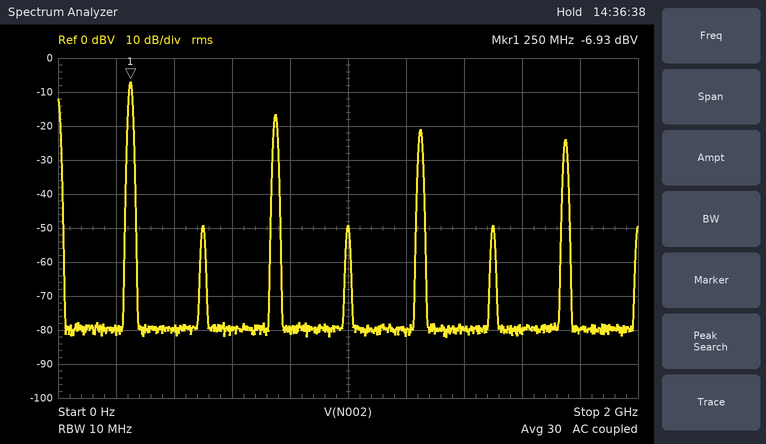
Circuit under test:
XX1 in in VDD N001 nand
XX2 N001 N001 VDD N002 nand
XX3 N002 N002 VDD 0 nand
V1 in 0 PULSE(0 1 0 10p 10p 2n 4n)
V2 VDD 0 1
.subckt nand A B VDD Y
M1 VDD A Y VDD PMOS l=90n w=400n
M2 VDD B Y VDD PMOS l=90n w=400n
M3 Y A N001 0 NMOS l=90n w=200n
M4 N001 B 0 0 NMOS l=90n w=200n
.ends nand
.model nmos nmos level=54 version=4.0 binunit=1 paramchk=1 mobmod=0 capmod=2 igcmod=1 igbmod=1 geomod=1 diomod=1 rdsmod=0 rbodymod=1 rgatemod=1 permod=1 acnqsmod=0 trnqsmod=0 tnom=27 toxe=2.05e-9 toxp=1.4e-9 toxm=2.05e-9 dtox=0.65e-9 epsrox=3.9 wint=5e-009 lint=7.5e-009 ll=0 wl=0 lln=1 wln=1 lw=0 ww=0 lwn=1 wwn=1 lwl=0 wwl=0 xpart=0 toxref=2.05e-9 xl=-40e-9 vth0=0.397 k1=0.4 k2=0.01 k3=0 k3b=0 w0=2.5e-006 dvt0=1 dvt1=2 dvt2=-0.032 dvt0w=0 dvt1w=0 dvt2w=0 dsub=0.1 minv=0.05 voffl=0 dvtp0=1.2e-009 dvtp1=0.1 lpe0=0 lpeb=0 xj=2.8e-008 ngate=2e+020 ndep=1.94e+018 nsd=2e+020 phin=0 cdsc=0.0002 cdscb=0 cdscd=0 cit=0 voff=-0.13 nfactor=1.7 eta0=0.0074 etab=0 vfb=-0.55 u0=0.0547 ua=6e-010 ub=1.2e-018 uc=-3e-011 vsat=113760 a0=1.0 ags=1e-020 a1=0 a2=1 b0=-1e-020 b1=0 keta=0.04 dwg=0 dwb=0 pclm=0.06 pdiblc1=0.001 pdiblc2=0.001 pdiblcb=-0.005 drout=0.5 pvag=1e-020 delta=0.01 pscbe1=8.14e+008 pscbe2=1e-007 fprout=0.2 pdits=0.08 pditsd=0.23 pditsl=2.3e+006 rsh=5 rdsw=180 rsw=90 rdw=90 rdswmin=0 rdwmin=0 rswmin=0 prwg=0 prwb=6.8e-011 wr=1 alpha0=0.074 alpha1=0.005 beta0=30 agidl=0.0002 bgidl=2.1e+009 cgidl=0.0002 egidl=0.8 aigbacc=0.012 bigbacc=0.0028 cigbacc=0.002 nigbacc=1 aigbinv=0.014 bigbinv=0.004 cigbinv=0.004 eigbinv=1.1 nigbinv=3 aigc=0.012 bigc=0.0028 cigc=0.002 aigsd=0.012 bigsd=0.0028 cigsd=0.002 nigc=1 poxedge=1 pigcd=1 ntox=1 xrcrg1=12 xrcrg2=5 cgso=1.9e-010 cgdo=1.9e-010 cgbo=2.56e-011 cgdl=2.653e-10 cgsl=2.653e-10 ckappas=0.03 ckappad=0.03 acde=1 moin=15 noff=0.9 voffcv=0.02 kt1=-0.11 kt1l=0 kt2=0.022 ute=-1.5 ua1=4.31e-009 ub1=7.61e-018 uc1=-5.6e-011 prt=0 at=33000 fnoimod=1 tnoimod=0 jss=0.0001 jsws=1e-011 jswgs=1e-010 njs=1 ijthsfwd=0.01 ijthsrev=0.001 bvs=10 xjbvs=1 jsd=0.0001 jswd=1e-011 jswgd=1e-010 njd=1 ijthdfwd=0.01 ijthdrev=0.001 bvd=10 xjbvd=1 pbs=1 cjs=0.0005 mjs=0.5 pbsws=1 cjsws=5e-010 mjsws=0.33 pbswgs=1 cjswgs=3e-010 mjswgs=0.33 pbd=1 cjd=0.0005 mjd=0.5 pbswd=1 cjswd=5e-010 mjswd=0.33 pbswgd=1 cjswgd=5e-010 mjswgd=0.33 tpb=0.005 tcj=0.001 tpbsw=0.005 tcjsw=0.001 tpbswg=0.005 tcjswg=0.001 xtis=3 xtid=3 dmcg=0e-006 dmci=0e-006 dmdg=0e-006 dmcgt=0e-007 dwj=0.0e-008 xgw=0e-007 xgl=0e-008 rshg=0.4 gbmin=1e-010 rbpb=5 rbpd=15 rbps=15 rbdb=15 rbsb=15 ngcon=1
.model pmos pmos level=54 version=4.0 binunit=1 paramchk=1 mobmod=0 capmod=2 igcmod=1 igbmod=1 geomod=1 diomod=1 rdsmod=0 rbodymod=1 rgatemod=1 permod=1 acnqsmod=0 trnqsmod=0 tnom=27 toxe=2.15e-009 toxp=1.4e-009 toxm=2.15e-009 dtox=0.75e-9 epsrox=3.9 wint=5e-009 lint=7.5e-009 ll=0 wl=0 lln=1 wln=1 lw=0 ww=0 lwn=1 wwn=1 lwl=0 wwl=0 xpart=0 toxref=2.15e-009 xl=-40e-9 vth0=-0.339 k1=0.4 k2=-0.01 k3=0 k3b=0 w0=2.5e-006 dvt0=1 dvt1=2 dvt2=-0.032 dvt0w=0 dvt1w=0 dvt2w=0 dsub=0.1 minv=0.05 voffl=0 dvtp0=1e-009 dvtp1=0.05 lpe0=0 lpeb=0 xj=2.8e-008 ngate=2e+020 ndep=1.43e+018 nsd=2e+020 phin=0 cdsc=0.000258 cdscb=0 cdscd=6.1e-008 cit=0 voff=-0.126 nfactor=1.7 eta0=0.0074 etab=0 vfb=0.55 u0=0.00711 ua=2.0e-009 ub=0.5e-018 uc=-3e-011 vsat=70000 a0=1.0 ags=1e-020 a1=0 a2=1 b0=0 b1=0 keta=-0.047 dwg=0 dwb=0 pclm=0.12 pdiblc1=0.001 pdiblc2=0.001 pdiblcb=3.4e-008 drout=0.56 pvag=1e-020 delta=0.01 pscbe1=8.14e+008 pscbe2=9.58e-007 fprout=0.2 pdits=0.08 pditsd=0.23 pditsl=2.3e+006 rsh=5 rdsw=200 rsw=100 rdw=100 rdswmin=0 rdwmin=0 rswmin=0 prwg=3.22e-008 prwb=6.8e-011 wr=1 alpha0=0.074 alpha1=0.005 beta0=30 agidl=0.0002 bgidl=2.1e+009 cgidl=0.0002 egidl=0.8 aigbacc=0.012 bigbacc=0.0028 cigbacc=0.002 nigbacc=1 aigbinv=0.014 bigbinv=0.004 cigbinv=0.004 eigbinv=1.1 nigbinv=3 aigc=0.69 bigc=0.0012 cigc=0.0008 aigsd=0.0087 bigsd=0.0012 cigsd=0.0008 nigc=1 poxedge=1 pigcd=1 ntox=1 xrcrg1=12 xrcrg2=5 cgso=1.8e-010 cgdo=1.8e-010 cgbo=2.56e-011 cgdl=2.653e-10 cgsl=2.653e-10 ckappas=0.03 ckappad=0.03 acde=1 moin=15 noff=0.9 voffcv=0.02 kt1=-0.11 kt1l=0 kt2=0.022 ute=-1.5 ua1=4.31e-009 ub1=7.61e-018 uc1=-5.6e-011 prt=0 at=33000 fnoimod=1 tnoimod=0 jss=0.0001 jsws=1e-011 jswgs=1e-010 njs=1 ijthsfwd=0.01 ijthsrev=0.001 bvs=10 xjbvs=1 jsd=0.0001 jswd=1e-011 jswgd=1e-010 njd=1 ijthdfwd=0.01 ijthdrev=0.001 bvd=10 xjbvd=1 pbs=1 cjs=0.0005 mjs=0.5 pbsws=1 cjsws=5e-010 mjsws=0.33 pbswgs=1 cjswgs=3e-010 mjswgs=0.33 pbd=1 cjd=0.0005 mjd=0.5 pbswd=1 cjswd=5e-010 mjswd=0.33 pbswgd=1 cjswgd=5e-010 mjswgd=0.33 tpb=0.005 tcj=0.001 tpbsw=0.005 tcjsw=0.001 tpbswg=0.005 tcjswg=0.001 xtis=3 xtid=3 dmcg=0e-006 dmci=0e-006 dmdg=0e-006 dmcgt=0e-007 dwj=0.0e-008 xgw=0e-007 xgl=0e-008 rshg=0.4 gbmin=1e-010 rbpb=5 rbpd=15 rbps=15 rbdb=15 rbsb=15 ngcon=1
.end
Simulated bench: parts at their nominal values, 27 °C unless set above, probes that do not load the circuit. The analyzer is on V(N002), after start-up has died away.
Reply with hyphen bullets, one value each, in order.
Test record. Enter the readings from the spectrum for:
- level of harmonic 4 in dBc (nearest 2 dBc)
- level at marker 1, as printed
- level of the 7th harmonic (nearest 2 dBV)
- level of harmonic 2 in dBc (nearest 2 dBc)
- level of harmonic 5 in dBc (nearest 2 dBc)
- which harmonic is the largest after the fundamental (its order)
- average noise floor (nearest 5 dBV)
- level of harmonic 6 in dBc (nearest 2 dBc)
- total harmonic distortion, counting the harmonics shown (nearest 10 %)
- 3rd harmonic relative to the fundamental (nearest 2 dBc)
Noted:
- -42 dBc
- -6.93 dBV
- -24 dBV
- -42 dBc
- -14 dBc
- 3
- -80 dBV
- -42 dBc
- 40 %
- -10 dBc
